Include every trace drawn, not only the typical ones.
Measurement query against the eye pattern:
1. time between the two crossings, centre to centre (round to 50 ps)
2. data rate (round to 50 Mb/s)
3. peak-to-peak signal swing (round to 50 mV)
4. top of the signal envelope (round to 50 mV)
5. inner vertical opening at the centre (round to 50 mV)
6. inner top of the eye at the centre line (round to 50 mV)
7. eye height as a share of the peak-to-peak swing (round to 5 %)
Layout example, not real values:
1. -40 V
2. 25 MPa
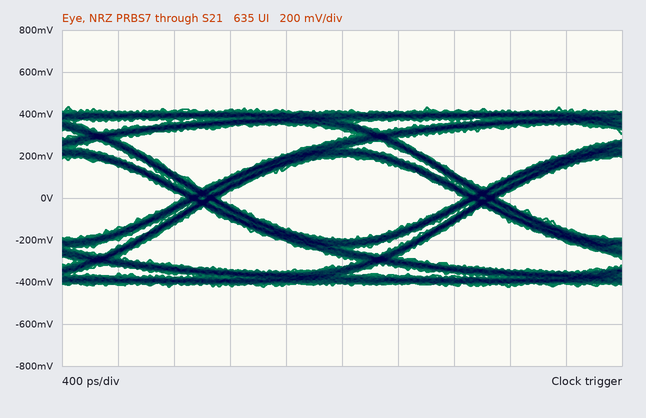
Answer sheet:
1. 2.00 ns
2. 500 Mb/s
3. 850 mV
4. 450 mV
5. 400 mV
6. 200 mV
7. 45 %
